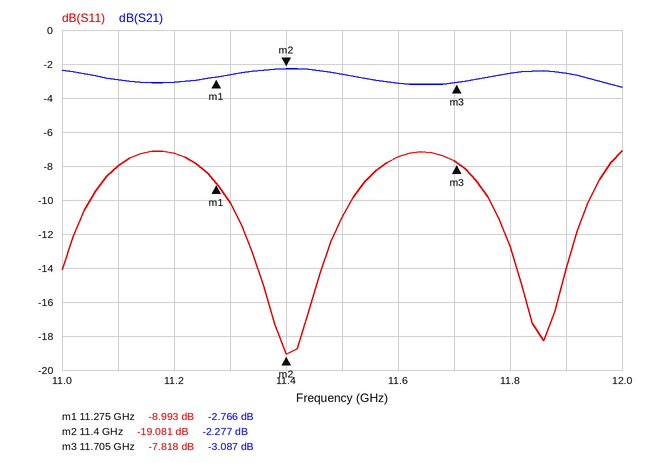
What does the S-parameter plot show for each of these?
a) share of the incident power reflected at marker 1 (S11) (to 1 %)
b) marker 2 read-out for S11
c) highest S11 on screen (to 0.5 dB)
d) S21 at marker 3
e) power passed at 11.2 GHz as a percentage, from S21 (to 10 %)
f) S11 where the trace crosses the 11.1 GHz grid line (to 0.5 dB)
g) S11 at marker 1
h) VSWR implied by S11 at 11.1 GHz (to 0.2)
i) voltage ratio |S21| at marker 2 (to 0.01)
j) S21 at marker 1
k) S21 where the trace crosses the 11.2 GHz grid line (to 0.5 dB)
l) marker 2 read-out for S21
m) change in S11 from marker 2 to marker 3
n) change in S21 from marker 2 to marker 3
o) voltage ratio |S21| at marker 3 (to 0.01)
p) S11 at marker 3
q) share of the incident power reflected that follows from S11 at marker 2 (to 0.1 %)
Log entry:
13 %
-19.081 dB
-7.0 dB
-3.087 dB
50 %
-8.0 dB
-8.993 dB
2.4
0.77
-2.766 dB
-3.0 dB
-2.277 dB
11.263 dB
-0.810 dB
0.70
-7.818 dB
1.2 %
